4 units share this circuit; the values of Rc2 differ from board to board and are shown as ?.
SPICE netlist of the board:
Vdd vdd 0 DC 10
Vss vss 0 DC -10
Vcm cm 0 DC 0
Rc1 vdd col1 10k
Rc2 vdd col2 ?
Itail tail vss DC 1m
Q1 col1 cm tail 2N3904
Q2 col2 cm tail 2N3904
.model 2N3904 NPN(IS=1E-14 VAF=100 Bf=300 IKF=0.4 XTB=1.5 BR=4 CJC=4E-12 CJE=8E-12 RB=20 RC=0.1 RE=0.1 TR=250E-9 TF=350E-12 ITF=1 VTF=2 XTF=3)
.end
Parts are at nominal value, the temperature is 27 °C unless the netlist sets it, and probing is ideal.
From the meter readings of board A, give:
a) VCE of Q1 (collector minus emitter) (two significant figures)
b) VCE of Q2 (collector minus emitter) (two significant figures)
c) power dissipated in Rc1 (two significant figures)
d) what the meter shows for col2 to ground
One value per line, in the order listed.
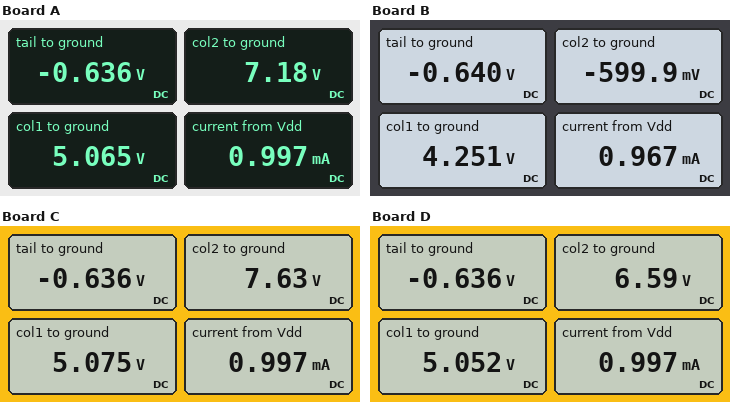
5.7 V
7.8 V
2.4 mW
7.18 V
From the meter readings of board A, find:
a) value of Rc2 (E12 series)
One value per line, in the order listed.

5.6 kΩ
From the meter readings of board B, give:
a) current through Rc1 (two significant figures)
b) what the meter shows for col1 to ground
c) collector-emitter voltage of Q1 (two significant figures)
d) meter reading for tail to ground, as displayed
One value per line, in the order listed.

570 µA
4.251 V
4.9 V
-0.640 V
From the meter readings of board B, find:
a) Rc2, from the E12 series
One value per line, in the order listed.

27 kΩ
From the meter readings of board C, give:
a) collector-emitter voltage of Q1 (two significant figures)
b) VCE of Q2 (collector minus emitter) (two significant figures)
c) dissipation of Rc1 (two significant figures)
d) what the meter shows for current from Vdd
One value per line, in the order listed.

5.7 V
8.3 V
2.4 mW
0.997 mA
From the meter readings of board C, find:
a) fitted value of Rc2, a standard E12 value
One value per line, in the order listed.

4.7 kΩ
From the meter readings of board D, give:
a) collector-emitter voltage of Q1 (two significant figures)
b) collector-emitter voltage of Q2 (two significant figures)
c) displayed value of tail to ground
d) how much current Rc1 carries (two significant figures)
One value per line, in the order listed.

5.7 V
7.2 V
-0.636 V
490 µA
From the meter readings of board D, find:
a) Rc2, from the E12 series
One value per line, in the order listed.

6.8 kΩ
